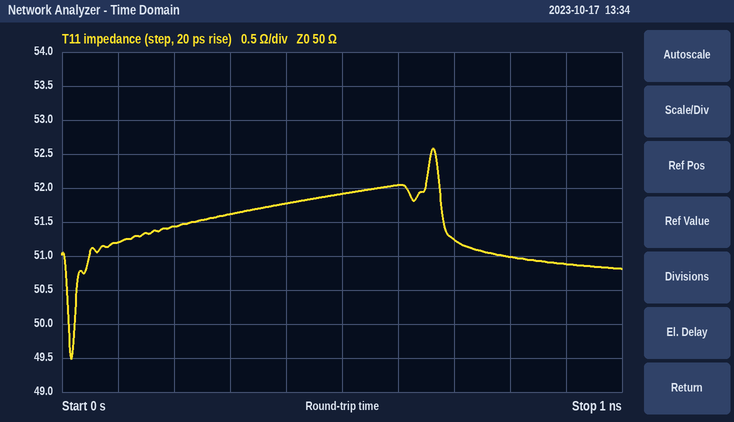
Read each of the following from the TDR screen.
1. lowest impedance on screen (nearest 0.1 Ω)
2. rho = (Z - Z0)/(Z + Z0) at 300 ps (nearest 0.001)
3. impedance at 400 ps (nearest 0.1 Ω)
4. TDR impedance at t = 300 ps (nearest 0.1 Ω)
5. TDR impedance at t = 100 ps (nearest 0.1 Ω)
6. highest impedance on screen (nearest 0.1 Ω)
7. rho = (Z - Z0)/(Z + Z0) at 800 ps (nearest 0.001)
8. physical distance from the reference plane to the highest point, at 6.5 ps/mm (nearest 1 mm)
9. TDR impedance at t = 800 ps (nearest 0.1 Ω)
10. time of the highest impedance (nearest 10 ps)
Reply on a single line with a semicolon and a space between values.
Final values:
49.5 Ω; +0.016; 51.8 Ω; 51.6 Ω; 51.2 Ω; 52.6 Ω; +0.010; 51 mm; 51.0 Ω; 660 ps
